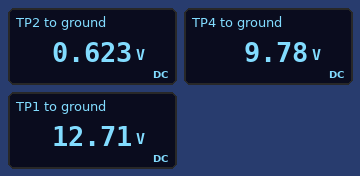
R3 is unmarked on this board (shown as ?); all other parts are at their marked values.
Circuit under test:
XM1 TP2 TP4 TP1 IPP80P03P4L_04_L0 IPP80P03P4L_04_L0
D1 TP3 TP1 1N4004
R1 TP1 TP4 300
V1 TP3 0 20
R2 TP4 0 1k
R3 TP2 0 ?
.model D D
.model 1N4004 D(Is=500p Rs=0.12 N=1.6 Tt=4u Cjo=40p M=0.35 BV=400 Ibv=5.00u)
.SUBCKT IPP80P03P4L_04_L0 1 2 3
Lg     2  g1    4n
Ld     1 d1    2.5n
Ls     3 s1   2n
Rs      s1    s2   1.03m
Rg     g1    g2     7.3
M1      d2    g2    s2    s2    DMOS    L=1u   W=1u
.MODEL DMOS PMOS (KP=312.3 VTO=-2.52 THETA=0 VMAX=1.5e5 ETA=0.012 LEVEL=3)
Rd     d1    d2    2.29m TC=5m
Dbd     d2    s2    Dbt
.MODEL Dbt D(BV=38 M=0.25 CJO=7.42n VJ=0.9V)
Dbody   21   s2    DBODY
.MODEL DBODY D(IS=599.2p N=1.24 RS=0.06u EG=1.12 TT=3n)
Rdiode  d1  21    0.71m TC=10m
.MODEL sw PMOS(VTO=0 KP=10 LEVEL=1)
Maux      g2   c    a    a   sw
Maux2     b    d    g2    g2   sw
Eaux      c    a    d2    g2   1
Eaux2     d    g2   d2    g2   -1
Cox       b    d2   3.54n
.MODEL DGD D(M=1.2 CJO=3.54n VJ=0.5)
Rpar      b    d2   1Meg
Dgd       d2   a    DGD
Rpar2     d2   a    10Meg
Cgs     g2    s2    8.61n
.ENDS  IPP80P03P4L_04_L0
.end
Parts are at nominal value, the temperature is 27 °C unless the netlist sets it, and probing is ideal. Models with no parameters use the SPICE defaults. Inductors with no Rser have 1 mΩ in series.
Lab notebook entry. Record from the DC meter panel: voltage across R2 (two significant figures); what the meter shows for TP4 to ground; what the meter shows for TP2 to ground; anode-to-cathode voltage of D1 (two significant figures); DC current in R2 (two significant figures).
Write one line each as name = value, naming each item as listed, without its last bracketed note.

voltage across R2 = 9.8 V
what the meter shows for TP4 to ground = 9.78 V
what the meter shows for TP2 to ground = 0.623 V
anode-to-cathode voltage of D1 = 7.3 V
DC current in R2 = 9.8 mA
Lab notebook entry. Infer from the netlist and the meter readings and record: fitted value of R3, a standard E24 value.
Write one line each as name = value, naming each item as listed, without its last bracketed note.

fitted value of R3, a standard E24 value = 0.012 Ω
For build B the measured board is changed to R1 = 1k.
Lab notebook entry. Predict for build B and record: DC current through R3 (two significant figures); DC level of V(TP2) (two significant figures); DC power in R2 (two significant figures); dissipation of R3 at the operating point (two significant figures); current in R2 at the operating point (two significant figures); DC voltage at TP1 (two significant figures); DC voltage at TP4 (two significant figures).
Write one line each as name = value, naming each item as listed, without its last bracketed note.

DC current through R3 = 99 A
DC level of V(TP2) = 1.2 V
DC power in R2 = 12 mW
dissipation of R3 at the operating point = 120 W
current in R2 at the operating point = 3.5 mA
DC voltage at TP1 = 7.0 V
DC voltage at TP4 = 3.5 V
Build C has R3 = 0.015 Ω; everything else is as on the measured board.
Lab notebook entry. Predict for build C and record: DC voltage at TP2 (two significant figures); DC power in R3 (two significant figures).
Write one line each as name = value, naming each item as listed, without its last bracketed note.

DC voltage at TP2 = 780 mV
DC power in R3 = 40 W
